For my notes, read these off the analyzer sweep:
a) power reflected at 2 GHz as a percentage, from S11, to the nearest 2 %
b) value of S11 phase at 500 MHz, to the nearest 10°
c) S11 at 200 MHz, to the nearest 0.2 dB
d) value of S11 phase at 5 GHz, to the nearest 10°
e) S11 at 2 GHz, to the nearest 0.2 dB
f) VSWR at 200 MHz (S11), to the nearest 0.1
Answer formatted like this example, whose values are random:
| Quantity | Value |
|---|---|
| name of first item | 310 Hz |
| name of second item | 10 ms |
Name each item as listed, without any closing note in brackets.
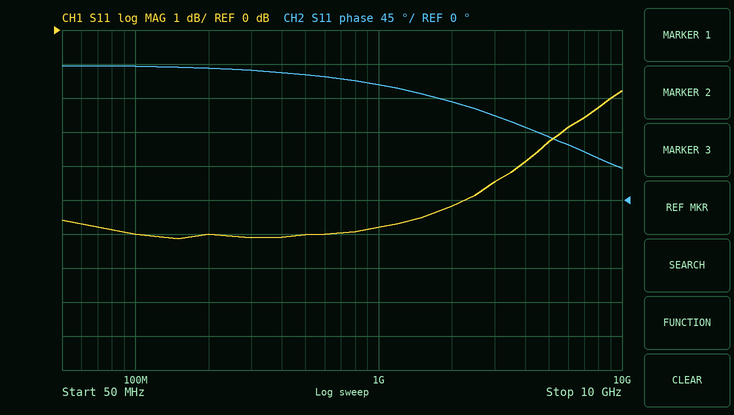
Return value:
| Quantity | Value |
|---|---|
| power reflected at 2 GHz as a percentage, from S11, to the nearest 2 % | 30 % |
| value of S11 phase at 500 MHz, to the nearest 10° | 170° |
| S11 at 200 MHz, to the nearest 0.2 dB | -6.0 dB |
| value of S11 phase at 5 GHz, to the nearest 10° | 80° |
| S11 at 2 GHz, to the nearest 0.2 dB | -5.2 dB |
| VSWR at 200 MHz (S11), to the nearest 0.1 | 3.0 |
